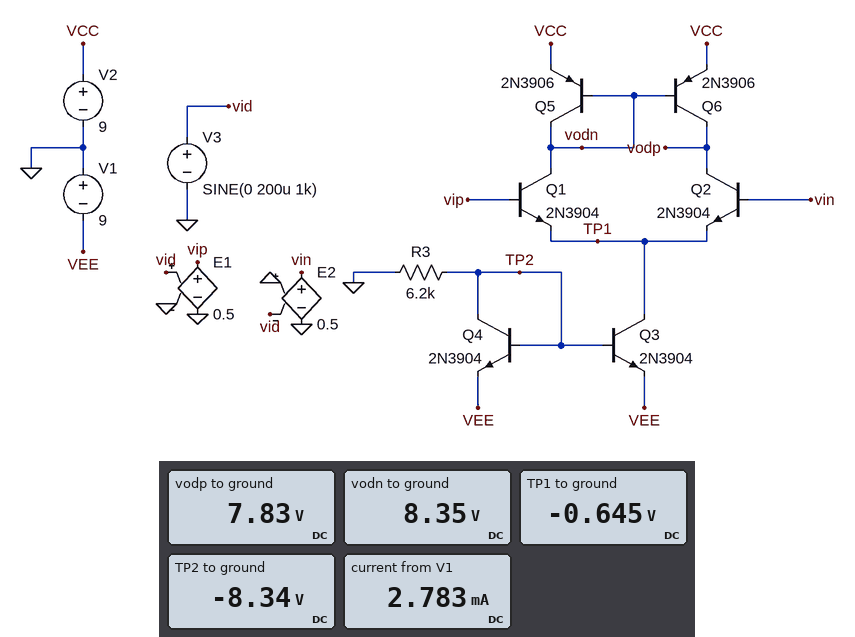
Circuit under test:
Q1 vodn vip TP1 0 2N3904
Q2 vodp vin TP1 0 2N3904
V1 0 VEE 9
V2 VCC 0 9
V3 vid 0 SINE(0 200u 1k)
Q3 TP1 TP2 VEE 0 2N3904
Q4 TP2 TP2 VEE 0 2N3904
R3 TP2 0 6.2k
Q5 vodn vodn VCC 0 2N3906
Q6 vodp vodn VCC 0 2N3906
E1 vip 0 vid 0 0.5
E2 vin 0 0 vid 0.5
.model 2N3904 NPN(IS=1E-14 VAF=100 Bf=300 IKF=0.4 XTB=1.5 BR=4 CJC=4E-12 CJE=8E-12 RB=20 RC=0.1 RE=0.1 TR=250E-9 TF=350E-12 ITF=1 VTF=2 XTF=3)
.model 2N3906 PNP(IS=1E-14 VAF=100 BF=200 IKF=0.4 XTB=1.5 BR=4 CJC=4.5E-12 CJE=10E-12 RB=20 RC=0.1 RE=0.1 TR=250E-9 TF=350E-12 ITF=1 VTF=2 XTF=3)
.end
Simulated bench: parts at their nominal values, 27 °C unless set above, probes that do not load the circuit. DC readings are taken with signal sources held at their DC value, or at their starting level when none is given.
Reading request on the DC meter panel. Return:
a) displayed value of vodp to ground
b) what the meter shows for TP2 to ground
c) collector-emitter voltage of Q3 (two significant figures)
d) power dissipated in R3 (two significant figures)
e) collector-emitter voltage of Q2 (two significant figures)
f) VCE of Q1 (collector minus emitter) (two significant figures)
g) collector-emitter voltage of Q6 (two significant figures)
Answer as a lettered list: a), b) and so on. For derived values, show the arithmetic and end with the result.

a) 7.83 V
b) -8.34 V
c) -645 mV - (-9 V) = 8.4 V
d) (0 V - (-8.34 V))^2 / 6.2 kΩ = 11 mW
e) 7.83 V - (-645 mV) = 8.5 V
f) 8.35 V - (-645 mV) = 9.0 V
g) 7.83 V - 9 V = -1.2 V
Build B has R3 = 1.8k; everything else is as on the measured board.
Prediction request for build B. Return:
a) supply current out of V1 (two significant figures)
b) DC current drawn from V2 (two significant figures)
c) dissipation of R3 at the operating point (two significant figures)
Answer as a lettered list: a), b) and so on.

a) 9.5 mA
b) 4.9 mA
c) 38 mW
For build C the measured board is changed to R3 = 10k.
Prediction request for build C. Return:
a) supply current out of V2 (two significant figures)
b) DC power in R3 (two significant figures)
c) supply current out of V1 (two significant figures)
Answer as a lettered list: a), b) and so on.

a) 890 µA
b) 7.0 mW
c) 1.7 mA
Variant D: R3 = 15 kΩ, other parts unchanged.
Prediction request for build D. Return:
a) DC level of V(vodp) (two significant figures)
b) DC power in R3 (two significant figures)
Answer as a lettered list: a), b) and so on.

a) 7.9 V
b) 4.7 mW
